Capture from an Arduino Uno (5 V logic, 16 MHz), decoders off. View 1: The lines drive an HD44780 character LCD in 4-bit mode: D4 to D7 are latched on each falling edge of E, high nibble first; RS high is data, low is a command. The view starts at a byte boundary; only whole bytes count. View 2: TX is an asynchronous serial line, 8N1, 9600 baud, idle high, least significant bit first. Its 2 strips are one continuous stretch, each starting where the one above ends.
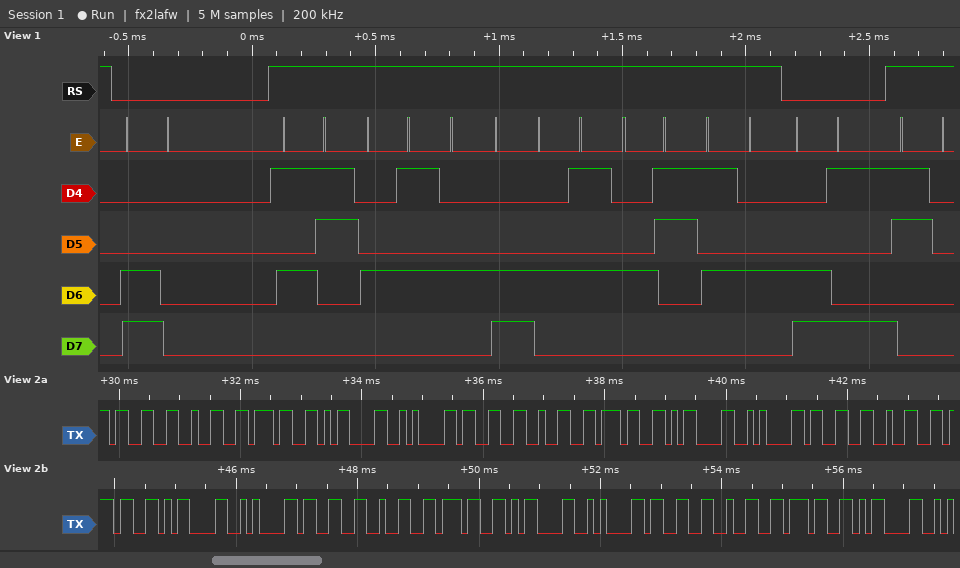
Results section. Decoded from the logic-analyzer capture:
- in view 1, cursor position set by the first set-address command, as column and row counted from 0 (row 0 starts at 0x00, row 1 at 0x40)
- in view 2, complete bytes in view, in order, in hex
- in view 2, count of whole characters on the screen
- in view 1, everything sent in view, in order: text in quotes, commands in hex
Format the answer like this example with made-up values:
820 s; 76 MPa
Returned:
column 0, row 1; 33 32 37 0D 0A 33 32 37 0D 0A 33 32 37 0D 0A 33 32 37 0D 0A 33 32 37 0D; 24; 0xC0 "SELECT" 0xC9 "0"
